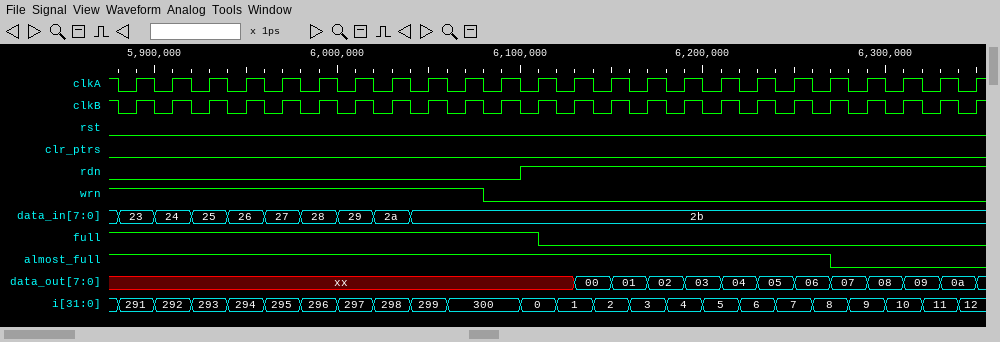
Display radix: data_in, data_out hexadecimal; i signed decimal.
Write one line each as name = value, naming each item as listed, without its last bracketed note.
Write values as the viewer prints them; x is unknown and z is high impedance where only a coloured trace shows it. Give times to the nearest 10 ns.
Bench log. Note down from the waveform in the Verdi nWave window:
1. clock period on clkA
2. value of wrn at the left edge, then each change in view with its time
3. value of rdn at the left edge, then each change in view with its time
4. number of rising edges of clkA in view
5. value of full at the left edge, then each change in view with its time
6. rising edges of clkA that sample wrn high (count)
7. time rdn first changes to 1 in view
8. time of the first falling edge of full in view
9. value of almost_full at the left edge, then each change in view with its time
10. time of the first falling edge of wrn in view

clock period on clkA = 20 ns
value of wrn at the left edge, then each change in view with its time = 1, 0 at 6080 ns
value of rdn at the left edge, then each change in view with its time = 0, 1 at 6100 ns
number of rising edges of clkA in view = 24
value of full at the left edge, then each change in view with its time = 1, 0 at 6110 ns
rising edges of clkA that sample wrn high = 10
time rdn first changes to 1 in view = 6100 ns
time of the first falling edge of full in view = 6110 ns
value of almost_full at the left edge, then each change in view with its time = 1, 0 at 6270 ns
time of the first falling edge of wrn in view = 6080 ns
